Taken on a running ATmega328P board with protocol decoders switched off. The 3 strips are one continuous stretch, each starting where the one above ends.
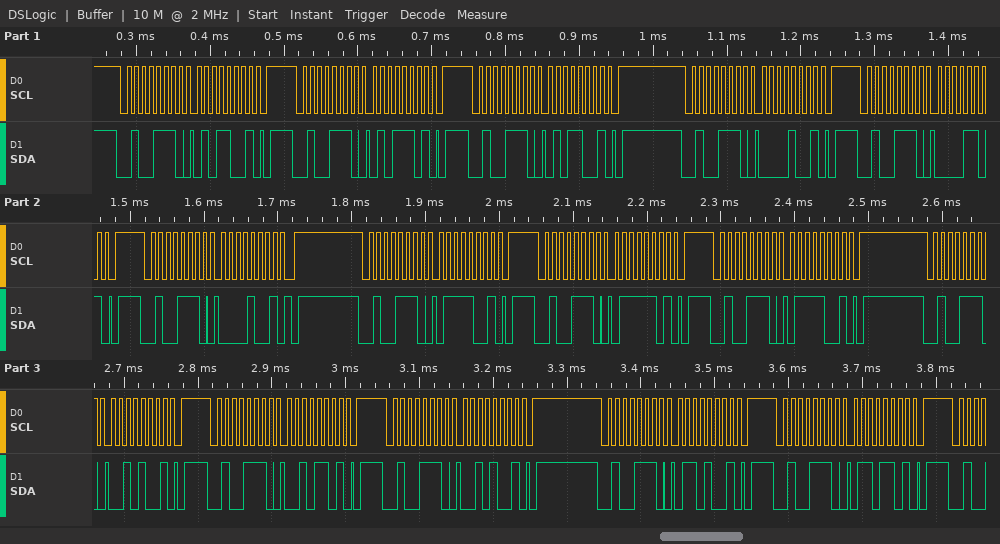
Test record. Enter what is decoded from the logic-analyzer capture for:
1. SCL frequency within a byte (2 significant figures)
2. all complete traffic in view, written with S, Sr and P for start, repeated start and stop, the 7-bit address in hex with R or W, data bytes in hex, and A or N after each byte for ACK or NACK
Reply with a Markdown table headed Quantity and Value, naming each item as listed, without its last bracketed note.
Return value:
| Quantity | Value |
|---|---|
| SCL frequency within a byte | 100 kHz |
| all complete traffic in view, written with S, Sr and P for start, repeated start and stop, the 7-bit address in hex with R or W, data bytes in hex, and A or N after each byte for ACK or NACK | S 27W A 59 A P S 27W A 5D A P S 27W A 59 A P S 27W A 09 A P S 27W A 0D A P S 27W A 09 A P S 27W A 79 A P S 27W A 7D A P S 27W A 79 A P S 27W A 29 A P S 27W A 2D A P S 27W A 29 A P S 27W A 69 A P S 27W A 6D A P |
